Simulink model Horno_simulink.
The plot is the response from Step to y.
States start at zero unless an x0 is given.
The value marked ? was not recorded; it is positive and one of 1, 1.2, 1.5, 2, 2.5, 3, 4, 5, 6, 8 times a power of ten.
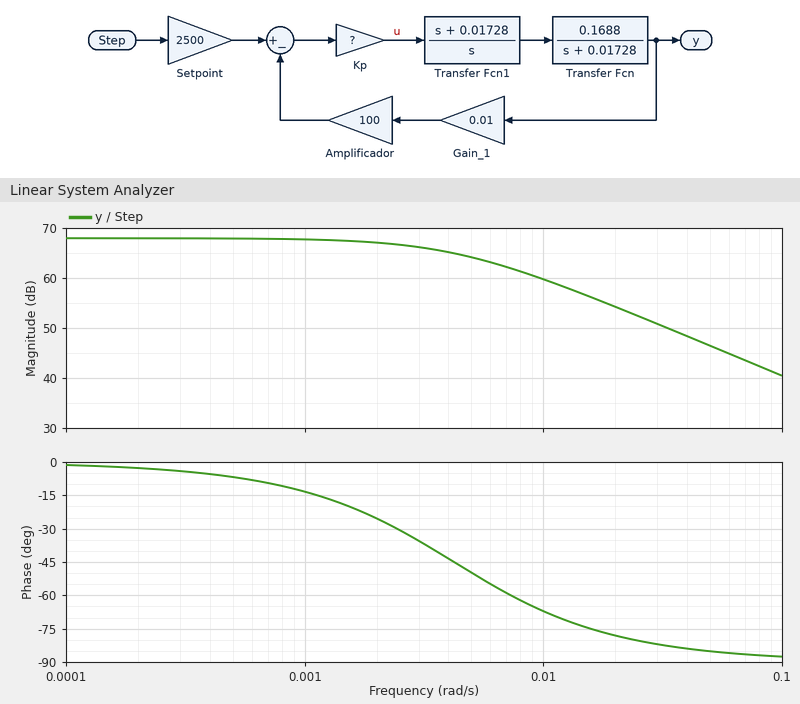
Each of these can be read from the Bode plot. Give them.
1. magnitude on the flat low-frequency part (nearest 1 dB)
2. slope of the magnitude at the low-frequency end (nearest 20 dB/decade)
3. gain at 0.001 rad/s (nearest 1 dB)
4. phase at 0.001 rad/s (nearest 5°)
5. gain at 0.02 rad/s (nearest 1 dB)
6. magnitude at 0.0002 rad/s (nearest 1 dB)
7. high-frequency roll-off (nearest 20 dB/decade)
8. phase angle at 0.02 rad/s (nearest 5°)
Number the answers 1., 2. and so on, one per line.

1. 68 dB
2. 0 dB/decade
3. 68 dB
4. -15°
5. 54 dB
6. 68 dB
7. -20 dB/decade
8. -80°
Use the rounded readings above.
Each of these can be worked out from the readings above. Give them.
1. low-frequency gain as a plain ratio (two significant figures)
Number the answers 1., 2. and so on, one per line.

1. 2500
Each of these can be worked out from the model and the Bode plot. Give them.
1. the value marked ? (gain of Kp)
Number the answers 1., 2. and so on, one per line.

1. 0.025
